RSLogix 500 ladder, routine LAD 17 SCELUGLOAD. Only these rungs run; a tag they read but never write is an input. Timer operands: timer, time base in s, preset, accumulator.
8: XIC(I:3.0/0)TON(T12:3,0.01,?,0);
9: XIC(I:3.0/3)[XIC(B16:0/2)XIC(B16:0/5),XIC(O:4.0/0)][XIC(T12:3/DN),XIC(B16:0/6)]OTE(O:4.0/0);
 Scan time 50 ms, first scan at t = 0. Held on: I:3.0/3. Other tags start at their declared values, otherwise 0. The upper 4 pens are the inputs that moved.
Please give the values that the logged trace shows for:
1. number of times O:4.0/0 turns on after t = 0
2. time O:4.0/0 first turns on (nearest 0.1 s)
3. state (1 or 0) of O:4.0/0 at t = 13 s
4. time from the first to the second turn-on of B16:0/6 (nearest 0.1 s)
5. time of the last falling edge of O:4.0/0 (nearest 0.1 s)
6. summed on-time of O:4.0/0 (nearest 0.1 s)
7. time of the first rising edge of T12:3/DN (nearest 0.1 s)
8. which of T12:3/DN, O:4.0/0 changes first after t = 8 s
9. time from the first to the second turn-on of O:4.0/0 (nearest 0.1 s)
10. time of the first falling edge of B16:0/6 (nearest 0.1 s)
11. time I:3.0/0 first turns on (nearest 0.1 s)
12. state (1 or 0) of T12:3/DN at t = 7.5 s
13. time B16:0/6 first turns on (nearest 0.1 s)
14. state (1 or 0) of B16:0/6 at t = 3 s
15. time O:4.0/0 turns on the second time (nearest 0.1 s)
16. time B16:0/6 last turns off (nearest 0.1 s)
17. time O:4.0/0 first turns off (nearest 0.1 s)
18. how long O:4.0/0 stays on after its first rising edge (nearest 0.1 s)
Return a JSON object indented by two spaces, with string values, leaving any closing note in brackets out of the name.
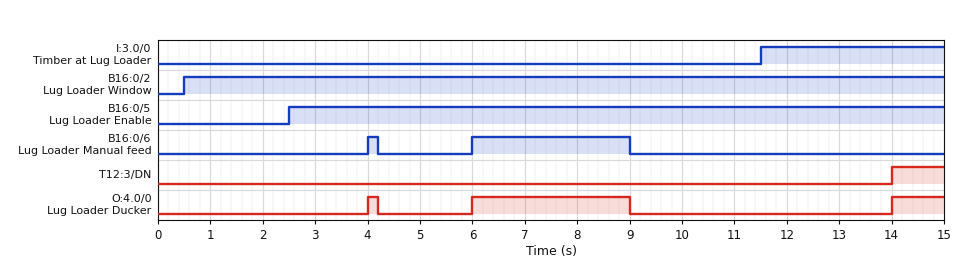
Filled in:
{
  "number of times O:4.0/0 turns on after t = 0": "3",
  "time O:4.0/0 first turns on": "4.0 s",
  "state (1 or 0) of O:4.0/0 at t = 13 s": "0",
  "time from the first to the second turn-on of B16:0/6": "2.0 s",
  "time of the last falling edge of O:4.0/0": "9.0 s",
  "summed on-time of O:4.0/0": "4.2 s",
  "time of the first rising edge of T12:3/DN": "14.0 s",
  "which of T12:3/DN, O:4.0/0 changes first after t = 8 s": "O:4.0/0",
  "time from the first to the second turn-on of O:4.0/0": "2.0 s",
  "time of the first falling edge of B16:0/6": "4.2 s",
  "time I:3.0/0 first turns on": "11.5 s",
  "state (1 or 0) of T12:3/DN at t = 7.5 s": "0",
  "time B16:0/6 first turns on": "4.0 s",
  "state (1 or 0) of B16:0/6 at t = 3 s": "0",
  "time O:4.0/0 turns on the second time": "6.0 s",
  "time B16:0/6 last turns off": "9.0 s",
  "time O:4.0/0 first turns off": "4.2 s",
  "how long O:4.0/0 stays on after its first rising edge": "0.2 s"
}
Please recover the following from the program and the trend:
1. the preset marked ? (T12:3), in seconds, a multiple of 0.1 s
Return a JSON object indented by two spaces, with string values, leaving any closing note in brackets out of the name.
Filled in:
{
  "the preset marked ? (T12:3), in seconds, a multiple of 0.1 s": "2.5 s"
}
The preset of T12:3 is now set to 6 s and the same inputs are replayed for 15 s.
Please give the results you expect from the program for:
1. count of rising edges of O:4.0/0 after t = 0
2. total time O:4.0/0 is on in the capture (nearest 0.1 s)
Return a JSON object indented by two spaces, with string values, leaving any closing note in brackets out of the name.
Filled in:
{
  "count of rising edges of O:4.0/0 after t = 0": "2",
  "total time O:4.0/0 is on in the capture": "3.2 s"
}
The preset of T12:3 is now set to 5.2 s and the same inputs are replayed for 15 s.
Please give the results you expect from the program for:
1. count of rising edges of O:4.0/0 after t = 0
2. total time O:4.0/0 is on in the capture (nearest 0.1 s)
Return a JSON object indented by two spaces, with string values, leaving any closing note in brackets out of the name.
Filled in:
{
  "count of rising edges of O:4.0/0 after t = 0": "2",
  "total time O:4.0/0 is on in the capture": "3.2 s"
}
